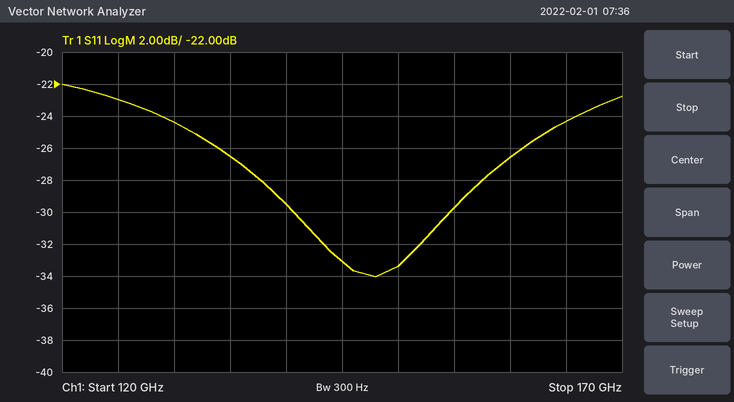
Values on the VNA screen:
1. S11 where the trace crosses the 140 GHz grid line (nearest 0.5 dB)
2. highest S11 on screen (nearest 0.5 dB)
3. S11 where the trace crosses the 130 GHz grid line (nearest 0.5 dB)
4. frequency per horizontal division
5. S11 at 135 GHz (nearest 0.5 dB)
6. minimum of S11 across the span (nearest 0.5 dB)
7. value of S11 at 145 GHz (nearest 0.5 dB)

-29.5 dB
-22.0 dB
-24.5 dB
5 GHz
-26.5 dB
-34.0 dB
-33.0 dB
